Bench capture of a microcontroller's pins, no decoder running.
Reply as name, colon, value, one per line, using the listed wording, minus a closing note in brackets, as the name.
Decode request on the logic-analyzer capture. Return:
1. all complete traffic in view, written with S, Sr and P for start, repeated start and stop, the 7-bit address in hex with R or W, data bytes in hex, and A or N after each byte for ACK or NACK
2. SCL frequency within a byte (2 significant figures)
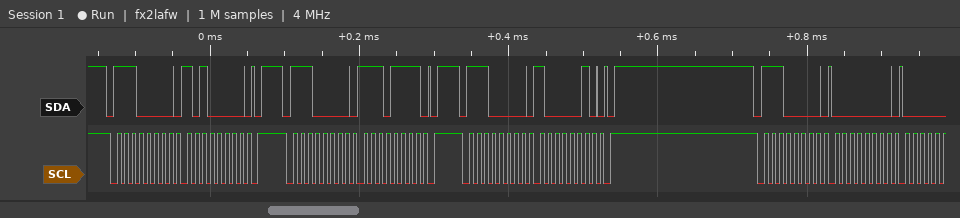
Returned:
all complete traffic in view, written with S, Sr and P for start, repeated start and stop, the 7-bit address in hex with R or W, data bytes in hex, and A or N after each byte for ACK or NACK: S 70W A A0 A P S 70W A EF A P S 70W A 82 A P S 70W A 00 A
SCL frequency within a byte: 100 kHz
